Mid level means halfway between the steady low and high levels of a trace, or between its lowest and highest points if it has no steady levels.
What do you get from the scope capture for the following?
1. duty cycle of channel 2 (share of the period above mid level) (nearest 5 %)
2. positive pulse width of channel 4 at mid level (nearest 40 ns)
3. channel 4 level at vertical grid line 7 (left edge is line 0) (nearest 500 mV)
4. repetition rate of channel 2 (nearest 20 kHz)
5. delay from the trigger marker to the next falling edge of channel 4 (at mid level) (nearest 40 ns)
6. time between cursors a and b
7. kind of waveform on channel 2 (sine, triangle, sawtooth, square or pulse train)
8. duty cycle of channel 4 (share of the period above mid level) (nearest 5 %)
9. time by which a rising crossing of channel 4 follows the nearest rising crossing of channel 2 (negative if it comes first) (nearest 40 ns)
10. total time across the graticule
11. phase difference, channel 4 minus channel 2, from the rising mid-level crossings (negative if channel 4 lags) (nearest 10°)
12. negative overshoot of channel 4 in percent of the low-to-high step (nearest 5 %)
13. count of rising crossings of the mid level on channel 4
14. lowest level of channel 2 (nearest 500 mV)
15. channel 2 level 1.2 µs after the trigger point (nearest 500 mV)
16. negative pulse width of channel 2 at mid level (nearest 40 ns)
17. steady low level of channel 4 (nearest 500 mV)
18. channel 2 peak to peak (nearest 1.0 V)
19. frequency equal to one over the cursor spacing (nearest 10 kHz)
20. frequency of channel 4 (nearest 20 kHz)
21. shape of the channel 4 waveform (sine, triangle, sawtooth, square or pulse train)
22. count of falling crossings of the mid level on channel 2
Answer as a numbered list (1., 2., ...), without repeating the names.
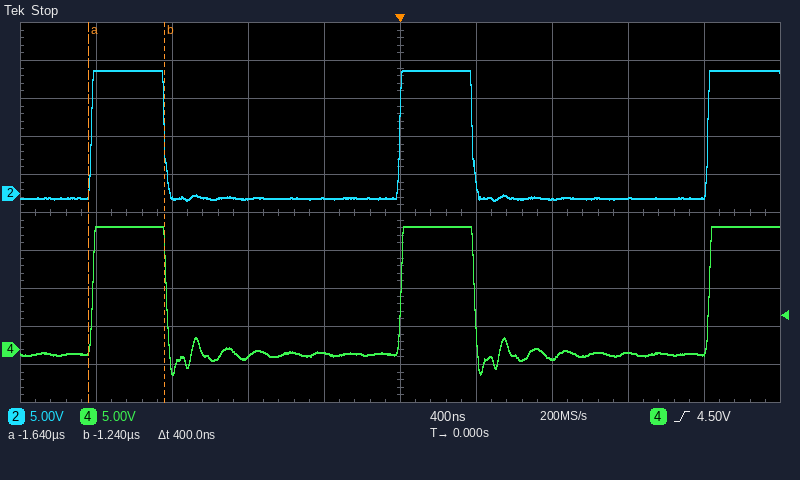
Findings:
1. 25 %
2. 400 ns
3. -1.0 V
4. 620 kHz
5. 400 ns
6. 400 ns
7. pulse train
8. 25 %
9. 0 ns
10. 4 µs
11. 0°
12. 15 %
13. 3
14. -1.0 V
15. -500 mV
16. 1.24 µs
17. -500 mV
18. 17.0 V
19. 2.50 MHz
20. 620 kHz
21. pulse train
22. 2
